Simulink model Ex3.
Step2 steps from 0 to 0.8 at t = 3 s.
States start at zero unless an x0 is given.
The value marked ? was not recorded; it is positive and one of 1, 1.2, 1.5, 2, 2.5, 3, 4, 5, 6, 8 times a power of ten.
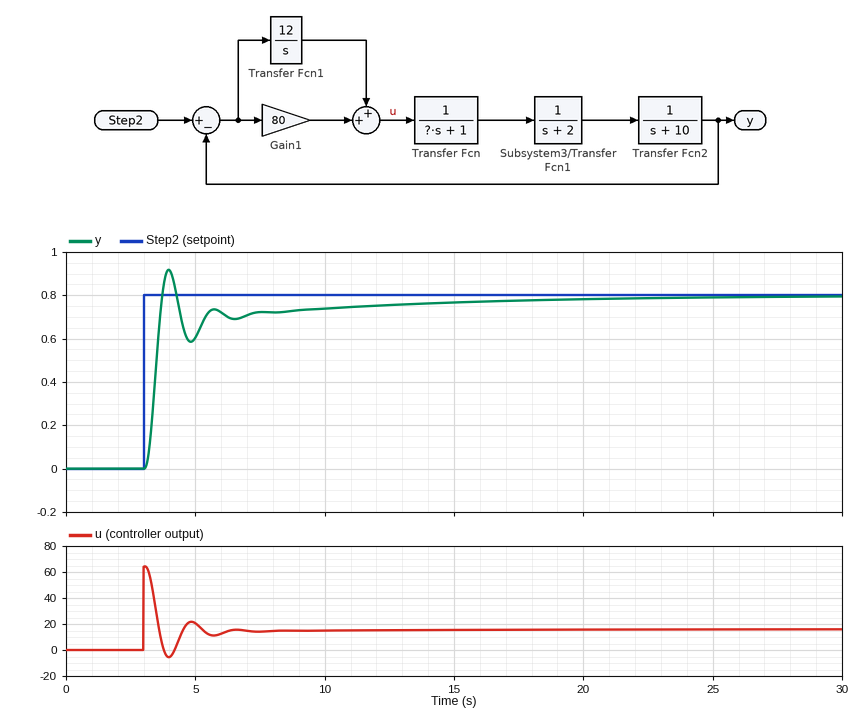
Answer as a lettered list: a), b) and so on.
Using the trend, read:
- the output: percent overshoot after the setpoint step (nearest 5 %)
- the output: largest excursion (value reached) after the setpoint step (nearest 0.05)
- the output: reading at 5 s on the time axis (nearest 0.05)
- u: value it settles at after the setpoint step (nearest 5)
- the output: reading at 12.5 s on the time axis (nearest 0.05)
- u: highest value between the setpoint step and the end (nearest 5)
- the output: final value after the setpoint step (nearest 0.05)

a) 15 %
b) 0.90
c) 0.60
d) 15
e) 0.75
f) 65
g) 0.80
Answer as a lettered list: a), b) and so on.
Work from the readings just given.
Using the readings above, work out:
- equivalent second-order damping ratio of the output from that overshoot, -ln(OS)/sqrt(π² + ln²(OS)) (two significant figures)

a) 0.52
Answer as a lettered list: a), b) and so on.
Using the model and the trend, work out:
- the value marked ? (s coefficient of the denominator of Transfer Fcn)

a) 0.6
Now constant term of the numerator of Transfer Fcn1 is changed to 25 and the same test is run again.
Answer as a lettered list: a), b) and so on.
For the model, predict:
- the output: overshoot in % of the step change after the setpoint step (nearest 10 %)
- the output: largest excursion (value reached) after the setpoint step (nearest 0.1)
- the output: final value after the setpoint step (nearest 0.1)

a) 20 %
b) 1.0
c) 0.8
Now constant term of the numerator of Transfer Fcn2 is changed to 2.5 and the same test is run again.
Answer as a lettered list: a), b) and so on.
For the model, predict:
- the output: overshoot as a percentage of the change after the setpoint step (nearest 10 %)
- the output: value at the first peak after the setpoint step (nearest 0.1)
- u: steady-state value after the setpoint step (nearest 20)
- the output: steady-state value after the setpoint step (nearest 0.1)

a) 60 %
b) 1.3
c) 0
d) 0.8
